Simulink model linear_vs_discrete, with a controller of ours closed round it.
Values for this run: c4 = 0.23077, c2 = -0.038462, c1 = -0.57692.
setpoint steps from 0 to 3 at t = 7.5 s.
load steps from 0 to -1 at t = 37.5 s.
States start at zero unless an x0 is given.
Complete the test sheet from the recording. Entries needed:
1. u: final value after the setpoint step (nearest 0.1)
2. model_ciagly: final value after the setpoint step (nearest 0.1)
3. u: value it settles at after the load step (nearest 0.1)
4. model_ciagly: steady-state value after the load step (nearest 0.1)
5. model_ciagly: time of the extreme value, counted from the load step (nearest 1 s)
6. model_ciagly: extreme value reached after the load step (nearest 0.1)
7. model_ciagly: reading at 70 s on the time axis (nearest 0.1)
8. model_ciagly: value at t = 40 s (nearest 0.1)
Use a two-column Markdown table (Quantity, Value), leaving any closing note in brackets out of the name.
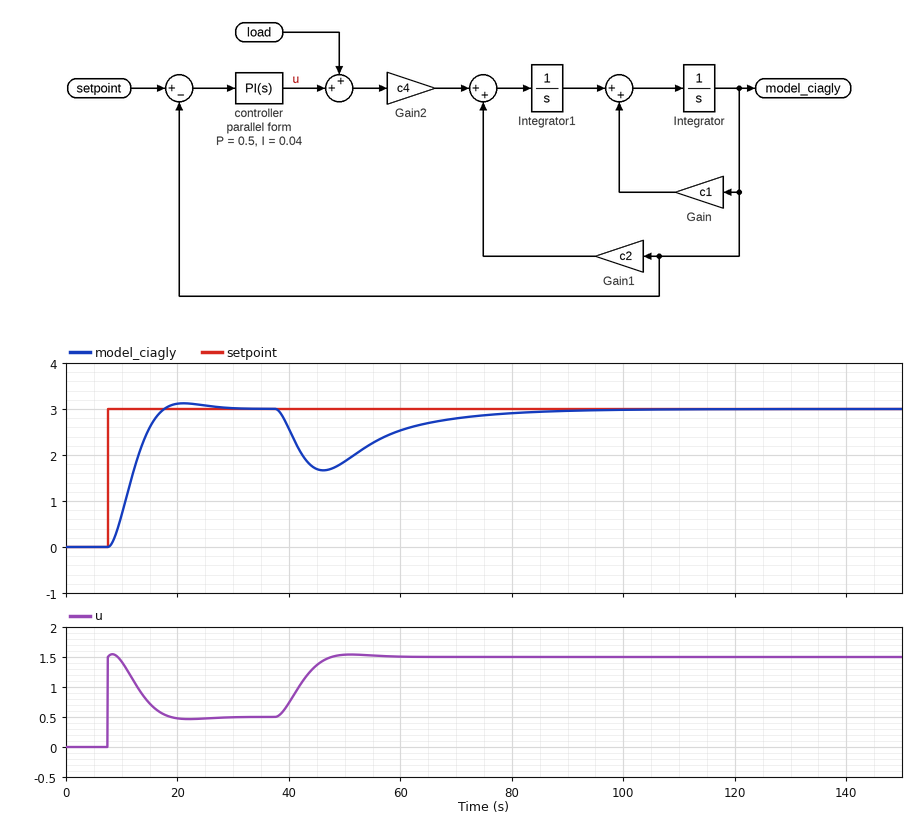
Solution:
| Quantity | Value |
|---|---|
| u: final value after the setpoint step | 0.5 |
| model_ciagly: final value after the setpoint step | 3.0 |
| u: value it settles at after the load step | 1.5 |
| model_ciagly: steady-state value after the load step | 3.0 |
| model_ciagly: time of the extreme value, counted from the load step | 9 s |
| model_ciagly: extreme value reached after the load step | 1.7 |
| model_ciagly: reading at 70 s on the time axis | 2.8 |
| model_ciagly: value at t = 40 s | 2.6 |
